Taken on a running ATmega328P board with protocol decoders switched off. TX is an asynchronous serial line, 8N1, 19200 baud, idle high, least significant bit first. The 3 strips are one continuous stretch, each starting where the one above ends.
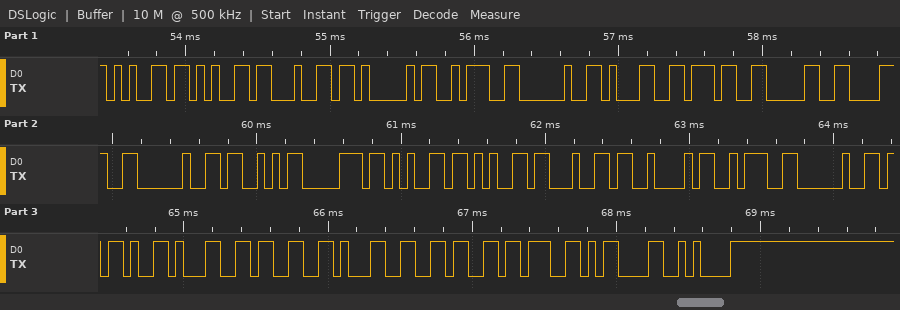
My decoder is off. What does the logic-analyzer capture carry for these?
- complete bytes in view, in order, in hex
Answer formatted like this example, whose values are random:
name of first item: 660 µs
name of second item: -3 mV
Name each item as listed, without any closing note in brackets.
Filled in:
complete bytes in view, in order, in hex: 65 65 64 41 3A 20 31 37 30 38 20 53 70 65 65 64 42 3A 20 2D 31 33 31 36 3B 0D 0A
